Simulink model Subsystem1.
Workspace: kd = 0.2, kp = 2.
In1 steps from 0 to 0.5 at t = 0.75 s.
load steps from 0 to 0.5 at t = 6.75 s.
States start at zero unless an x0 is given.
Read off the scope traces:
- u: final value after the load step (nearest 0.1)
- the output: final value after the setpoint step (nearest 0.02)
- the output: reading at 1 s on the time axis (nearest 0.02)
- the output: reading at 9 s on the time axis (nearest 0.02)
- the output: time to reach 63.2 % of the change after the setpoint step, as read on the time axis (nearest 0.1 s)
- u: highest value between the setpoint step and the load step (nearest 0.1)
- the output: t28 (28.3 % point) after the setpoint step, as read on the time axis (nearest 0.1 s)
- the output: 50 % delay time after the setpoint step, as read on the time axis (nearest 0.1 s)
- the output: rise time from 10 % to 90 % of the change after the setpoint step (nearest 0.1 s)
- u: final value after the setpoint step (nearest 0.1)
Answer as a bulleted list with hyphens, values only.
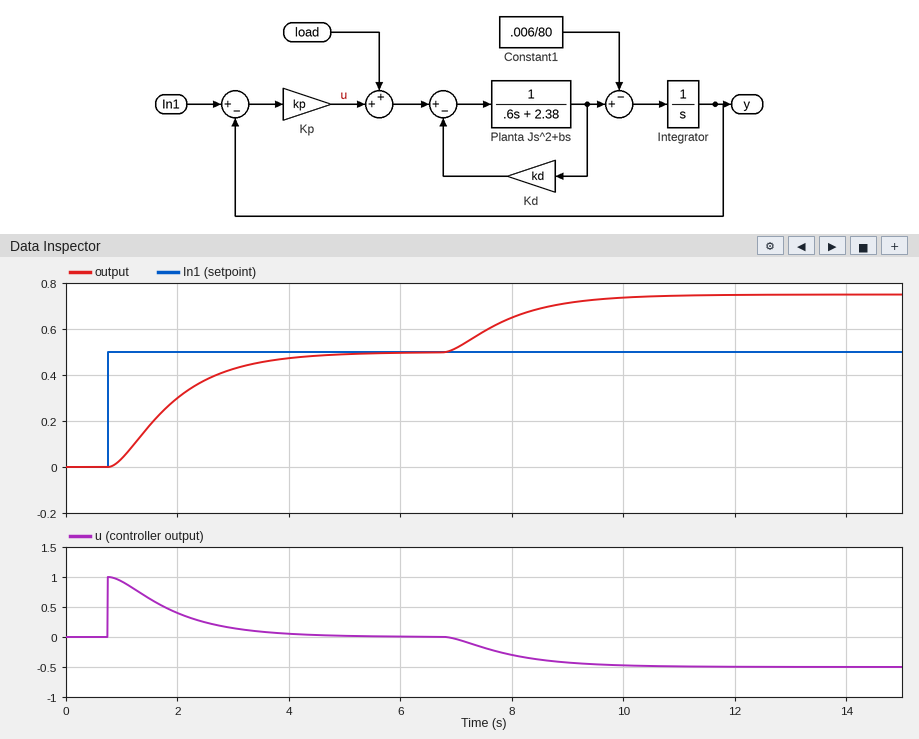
- -0.5
- 0.50
- 0.04
- 0.72
- 2.1 s
- 1.0
- 1.4 s
- 1.8 s
- 2.3 s
- 0.0
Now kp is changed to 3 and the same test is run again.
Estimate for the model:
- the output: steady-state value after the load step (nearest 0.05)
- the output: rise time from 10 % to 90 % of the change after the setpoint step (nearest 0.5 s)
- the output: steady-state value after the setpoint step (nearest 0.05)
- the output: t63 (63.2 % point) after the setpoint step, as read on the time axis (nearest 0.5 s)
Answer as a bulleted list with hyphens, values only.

- 0.65
- 1.5 s
- 0.50
- 1.5 s
